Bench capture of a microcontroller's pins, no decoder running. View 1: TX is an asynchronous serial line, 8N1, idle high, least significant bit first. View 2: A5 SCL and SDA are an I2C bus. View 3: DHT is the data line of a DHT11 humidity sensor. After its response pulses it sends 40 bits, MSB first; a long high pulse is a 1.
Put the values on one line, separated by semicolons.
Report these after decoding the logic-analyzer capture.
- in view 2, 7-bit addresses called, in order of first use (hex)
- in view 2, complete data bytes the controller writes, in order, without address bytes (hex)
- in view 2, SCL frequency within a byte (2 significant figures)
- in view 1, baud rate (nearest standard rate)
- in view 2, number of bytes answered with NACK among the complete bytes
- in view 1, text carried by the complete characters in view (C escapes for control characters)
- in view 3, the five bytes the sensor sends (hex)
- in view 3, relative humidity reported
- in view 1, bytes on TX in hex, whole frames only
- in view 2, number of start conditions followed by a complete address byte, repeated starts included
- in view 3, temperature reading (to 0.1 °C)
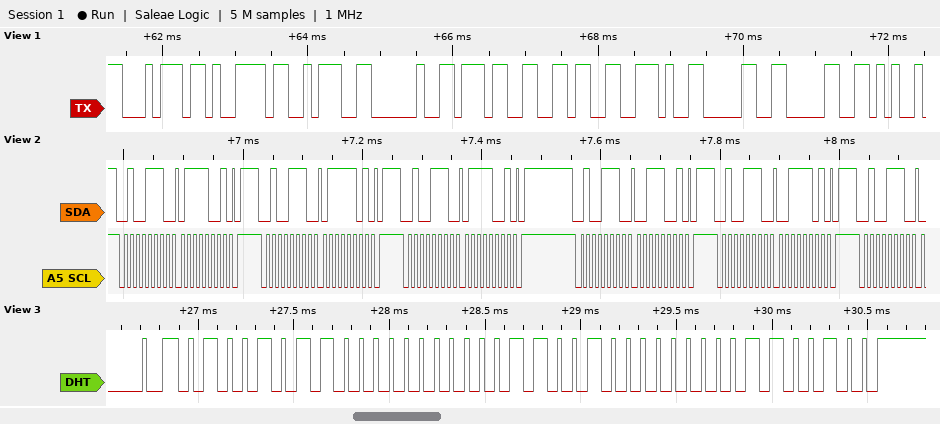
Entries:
0x27; 79 7D 79 39 3D; 100 kHz; 9600 baud; 0; "ty: 76.00"; 4B 00 19 00 64; 75 %; 74 79 3A 20 37 36 2E 30 30; 6; 25.0 °C
